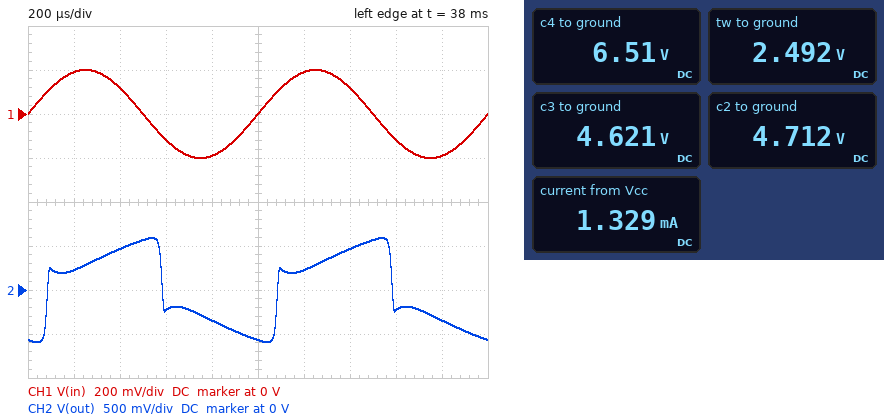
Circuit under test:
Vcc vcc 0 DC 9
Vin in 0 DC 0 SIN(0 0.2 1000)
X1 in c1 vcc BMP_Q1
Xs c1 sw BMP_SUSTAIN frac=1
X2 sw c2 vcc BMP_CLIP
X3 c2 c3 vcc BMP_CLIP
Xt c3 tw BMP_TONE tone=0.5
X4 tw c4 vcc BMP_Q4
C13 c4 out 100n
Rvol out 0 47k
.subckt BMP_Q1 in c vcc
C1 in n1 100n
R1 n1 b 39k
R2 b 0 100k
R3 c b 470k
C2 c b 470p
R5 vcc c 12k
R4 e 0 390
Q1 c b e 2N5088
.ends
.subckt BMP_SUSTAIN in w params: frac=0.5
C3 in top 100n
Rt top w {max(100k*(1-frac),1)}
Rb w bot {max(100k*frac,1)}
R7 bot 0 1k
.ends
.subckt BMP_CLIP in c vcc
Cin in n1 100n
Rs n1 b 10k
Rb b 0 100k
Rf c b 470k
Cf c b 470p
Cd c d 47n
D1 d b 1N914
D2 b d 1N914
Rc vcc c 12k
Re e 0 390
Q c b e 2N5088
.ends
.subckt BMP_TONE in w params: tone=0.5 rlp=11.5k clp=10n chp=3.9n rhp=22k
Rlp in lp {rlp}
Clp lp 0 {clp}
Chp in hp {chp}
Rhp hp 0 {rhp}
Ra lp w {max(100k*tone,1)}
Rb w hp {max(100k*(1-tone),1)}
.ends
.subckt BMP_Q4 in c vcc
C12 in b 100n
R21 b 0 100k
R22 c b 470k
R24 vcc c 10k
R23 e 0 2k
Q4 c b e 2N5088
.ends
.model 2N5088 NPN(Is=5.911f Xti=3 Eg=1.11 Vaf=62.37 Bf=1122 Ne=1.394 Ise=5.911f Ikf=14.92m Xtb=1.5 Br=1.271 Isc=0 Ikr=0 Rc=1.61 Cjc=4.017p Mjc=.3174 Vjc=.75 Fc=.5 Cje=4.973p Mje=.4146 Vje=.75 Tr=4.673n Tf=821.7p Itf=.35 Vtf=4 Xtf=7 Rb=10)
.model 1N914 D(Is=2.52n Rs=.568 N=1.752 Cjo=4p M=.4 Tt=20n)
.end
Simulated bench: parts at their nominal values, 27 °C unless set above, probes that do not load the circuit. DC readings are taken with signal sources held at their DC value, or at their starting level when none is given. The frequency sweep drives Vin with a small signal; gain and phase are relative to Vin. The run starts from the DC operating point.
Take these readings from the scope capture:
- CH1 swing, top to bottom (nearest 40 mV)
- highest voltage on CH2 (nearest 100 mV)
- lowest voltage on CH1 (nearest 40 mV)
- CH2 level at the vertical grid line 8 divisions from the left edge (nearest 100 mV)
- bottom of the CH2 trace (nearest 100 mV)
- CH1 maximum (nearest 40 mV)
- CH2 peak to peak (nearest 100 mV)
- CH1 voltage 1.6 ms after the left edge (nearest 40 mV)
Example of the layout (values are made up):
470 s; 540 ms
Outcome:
400 mV; 600 mV; -200 mV; -200 mV; -600 mV; 200 mV; 1.2 V; -120 mV
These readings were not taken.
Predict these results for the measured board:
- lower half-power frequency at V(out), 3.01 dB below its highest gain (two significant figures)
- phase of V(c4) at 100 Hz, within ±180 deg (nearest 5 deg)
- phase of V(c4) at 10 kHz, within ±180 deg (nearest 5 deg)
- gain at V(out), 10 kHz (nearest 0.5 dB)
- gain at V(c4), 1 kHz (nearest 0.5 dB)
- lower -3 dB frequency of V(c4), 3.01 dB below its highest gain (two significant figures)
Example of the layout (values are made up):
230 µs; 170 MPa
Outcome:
99 Hz; 85 deg; 140 deg; 16.0 dB; 51.5 dB; 93 Hz
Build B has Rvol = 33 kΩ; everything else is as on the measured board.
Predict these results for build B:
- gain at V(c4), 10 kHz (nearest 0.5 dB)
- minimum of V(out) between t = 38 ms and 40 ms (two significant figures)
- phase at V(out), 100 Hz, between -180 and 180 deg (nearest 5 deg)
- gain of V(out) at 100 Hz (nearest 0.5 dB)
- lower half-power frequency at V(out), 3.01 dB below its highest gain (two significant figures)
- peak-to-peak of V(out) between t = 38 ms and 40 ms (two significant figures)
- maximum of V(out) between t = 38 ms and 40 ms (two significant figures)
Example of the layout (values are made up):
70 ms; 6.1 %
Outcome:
15.5 dB; -560 mV; 110 deg; 54.0 dB; 100 Hz; 1.1 V; 550 mV
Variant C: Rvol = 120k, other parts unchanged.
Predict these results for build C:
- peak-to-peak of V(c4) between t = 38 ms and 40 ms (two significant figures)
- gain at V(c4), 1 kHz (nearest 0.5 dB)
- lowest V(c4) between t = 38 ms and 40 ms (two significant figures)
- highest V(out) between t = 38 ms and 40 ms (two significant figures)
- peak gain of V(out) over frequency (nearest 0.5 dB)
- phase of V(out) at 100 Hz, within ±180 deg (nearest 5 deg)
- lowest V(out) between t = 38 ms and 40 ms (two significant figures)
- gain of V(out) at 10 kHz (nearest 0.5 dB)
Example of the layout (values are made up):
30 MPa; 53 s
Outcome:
1.3 V; 52.5 dB; 5.8 V; 660 mV; 58.5 dB; 95 deg; -660 mV; 17.0 dB
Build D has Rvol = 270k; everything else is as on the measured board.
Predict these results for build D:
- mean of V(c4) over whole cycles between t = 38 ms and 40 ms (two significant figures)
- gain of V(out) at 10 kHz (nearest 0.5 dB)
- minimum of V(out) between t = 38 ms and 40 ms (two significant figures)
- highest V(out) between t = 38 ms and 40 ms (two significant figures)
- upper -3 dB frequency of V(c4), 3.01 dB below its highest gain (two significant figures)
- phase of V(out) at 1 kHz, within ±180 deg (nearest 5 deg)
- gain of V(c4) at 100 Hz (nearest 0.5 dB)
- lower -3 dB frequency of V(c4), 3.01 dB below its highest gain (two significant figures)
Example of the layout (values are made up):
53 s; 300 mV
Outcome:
6.5 V; 17.0 dB; -690 mV; 690 mV; 700 Hz; -90 deg; 56.0 dB; 95 Hz
